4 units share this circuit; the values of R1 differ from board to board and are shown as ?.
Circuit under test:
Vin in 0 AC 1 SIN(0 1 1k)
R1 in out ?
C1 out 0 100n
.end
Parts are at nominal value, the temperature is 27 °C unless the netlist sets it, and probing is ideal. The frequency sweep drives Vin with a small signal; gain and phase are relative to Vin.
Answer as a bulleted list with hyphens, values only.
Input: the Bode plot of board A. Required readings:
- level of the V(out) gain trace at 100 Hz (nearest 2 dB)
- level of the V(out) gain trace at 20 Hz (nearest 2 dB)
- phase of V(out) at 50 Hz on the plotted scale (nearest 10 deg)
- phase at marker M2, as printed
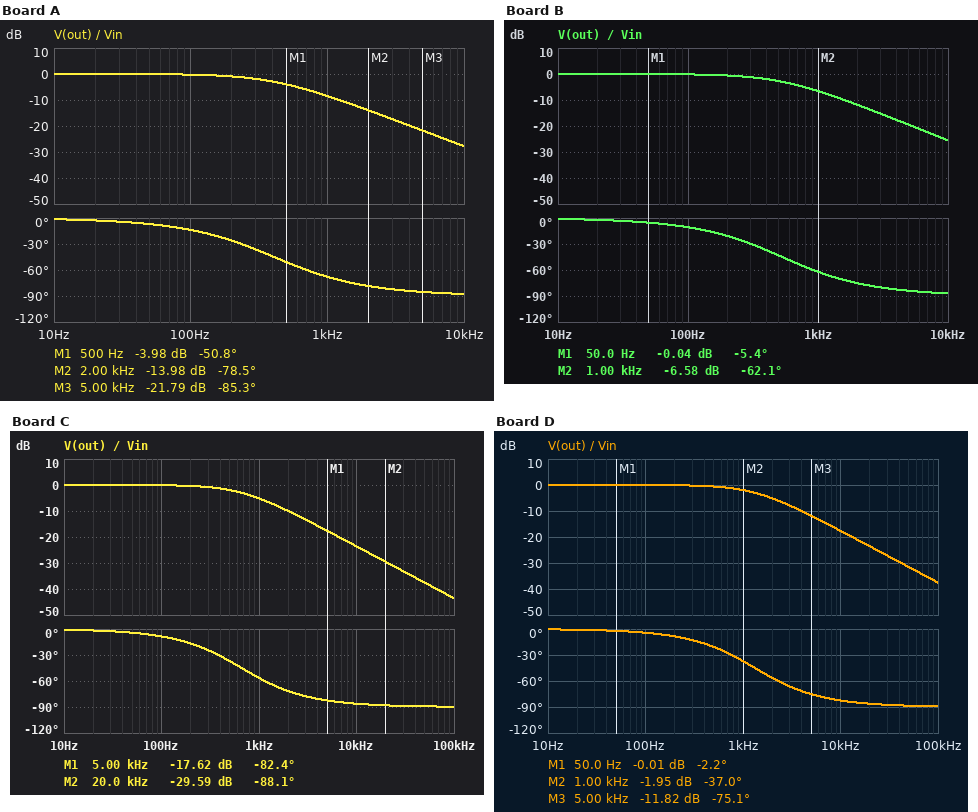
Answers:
- 0 dB
- 0 dB
- -10 deg
- -78.5 deg
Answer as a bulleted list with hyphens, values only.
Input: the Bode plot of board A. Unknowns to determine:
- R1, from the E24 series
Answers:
- 3.9 kΩ
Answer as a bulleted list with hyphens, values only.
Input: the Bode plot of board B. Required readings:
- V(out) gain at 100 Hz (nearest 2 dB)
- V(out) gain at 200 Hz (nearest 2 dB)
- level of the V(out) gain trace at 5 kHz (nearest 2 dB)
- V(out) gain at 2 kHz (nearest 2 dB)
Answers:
- 0 dB
- 0 dB
- -20 dB
- -12 dB
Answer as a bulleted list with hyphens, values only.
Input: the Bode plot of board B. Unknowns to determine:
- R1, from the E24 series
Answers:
- 3 kΩ
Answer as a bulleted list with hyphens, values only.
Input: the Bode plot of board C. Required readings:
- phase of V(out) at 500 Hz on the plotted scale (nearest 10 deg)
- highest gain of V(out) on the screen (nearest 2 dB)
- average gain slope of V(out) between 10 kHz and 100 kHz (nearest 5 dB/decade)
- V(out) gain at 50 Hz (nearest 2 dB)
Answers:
- -40 deg
- 0 dB
- -20 dB/decade
- 0 dB
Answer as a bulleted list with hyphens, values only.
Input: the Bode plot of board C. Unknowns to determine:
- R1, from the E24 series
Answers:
- 2.4 kΩ
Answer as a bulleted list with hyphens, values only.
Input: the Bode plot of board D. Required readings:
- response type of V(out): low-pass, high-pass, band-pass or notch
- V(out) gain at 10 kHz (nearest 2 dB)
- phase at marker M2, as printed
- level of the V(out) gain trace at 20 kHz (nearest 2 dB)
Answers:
- low-pass
- -18 dB
- -37.0 deg
- -24 dB
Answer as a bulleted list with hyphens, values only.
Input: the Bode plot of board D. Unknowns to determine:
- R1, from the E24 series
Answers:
- 1.2 kΩ
